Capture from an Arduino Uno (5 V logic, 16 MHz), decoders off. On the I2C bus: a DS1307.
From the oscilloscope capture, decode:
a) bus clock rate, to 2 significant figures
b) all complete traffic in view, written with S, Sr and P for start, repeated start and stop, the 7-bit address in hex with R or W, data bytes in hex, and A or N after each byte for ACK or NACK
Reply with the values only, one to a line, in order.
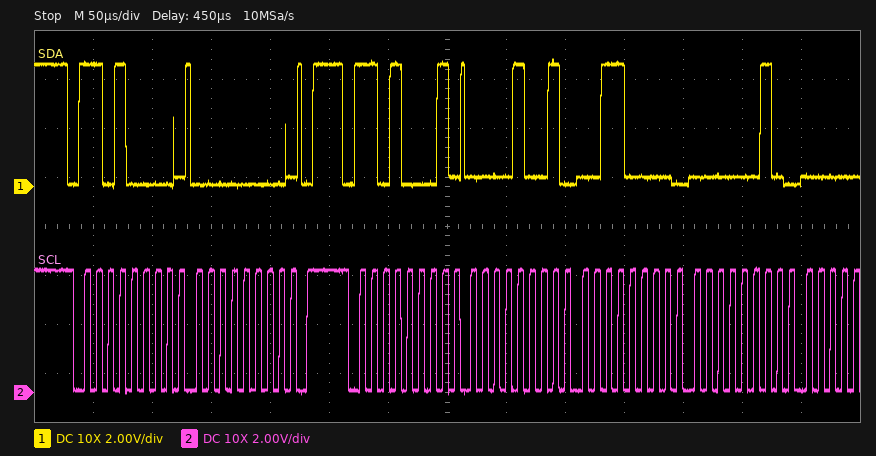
100 kHz
S 68W A 00 A P S 68R A 09 A 30 A 02 A
